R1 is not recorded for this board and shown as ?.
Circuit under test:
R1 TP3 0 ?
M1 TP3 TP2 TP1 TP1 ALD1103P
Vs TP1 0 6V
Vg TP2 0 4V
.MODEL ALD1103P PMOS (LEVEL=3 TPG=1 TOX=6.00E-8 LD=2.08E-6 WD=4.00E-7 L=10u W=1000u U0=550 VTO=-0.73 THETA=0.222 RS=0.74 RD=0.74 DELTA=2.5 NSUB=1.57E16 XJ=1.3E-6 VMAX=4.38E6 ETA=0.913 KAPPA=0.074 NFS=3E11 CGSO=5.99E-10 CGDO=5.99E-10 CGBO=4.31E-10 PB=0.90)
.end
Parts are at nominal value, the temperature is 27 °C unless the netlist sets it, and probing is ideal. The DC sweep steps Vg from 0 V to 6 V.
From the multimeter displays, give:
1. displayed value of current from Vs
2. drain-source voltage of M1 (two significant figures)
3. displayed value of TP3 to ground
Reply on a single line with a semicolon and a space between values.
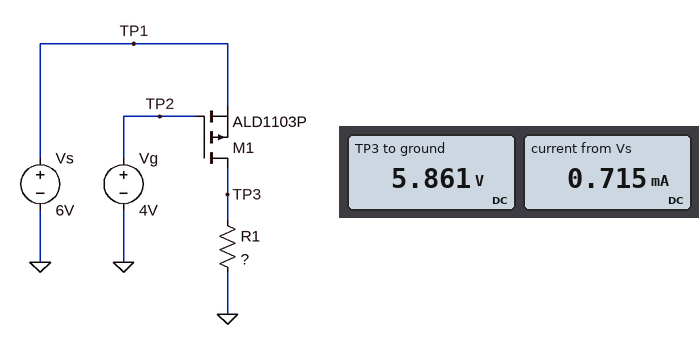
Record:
0.715 mA; -140 mV; 5.861 V
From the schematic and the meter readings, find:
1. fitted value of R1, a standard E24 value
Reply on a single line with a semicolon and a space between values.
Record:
8.2 kΩ
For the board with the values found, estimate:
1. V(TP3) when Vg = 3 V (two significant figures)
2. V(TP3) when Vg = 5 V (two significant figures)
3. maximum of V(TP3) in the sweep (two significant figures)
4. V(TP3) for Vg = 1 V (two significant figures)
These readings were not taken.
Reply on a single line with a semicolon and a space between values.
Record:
5.9 V; 1.8 V; 5.9 V; 5.9 V
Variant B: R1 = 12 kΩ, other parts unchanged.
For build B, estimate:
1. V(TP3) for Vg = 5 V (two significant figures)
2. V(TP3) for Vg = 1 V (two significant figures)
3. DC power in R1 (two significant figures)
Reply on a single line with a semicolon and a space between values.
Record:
2.5 V; 6.0 V; 2.9 mW
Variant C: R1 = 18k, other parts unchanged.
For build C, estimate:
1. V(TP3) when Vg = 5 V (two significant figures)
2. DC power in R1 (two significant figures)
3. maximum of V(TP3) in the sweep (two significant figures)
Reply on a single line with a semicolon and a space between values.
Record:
3.6 V; 2.0 mW; 6.0 V
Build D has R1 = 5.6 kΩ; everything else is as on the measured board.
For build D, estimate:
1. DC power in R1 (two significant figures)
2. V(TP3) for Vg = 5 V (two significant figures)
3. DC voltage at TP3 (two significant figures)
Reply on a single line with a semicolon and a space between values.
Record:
6.0 mW; 1.2 V; 5.8 V
